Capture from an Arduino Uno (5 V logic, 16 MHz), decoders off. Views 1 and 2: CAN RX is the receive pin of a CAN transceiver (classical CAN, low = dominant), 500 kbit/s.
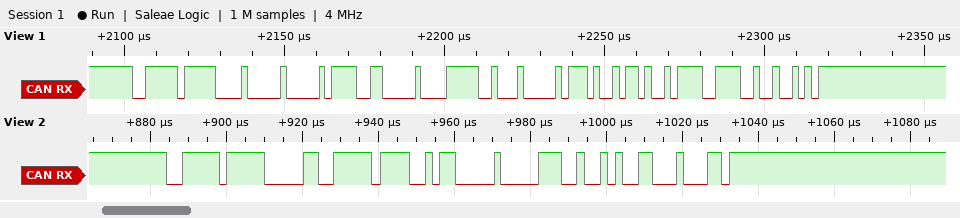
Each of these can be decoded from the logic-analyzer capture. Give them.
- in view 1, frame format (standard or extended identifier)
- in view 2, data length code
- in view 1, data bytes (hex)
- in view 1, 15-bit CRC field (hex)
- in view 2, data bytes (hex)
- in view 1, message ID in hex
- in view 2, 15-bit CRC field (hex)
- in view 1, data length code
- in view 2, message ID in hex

standard
4
00 F3 00 7D 10 3A 5A 5E
0x3C92
FF 96 00 64
0x3FF
0x5311
8
0x3FF
